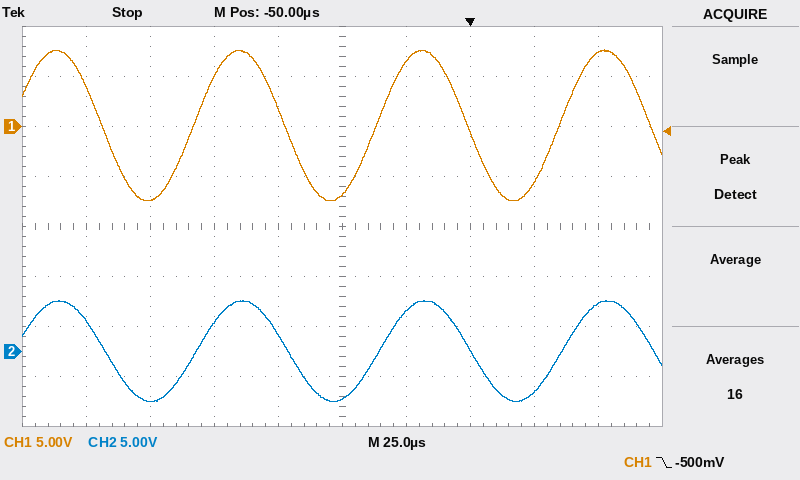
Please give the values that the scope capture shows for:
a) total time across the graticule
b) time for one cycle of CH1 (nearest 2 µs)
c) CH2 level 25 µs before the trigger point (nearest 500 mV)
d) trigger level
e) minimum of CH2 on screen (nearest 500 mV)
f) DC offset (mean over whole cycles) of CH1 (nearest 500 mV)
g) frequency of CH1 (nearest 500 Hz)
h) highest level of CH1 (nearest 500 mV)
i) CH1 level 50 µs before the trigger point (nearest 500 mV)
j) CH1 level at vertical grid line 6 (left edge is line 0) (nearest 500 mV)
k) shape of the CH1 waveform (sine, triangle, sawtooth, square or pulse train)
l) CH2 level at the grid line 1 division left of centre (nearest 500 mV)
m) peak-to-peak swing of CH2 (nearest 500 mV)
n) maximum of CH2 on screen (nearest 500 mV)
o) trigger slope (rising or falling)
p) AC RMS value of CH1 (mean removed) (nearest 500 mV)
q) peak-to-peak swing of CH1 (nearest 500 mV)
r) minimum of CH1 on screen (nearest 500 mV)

250 µs
72 µs
4.0 V
-500 mV
-5.0 V
0.0 V
14.0 kHz
7.5 V
-7.0 V
6.5 V
sine
1.5 V
10.0 V
5.0 V
falling
5.5 V
15.0 V
-7.5 V
